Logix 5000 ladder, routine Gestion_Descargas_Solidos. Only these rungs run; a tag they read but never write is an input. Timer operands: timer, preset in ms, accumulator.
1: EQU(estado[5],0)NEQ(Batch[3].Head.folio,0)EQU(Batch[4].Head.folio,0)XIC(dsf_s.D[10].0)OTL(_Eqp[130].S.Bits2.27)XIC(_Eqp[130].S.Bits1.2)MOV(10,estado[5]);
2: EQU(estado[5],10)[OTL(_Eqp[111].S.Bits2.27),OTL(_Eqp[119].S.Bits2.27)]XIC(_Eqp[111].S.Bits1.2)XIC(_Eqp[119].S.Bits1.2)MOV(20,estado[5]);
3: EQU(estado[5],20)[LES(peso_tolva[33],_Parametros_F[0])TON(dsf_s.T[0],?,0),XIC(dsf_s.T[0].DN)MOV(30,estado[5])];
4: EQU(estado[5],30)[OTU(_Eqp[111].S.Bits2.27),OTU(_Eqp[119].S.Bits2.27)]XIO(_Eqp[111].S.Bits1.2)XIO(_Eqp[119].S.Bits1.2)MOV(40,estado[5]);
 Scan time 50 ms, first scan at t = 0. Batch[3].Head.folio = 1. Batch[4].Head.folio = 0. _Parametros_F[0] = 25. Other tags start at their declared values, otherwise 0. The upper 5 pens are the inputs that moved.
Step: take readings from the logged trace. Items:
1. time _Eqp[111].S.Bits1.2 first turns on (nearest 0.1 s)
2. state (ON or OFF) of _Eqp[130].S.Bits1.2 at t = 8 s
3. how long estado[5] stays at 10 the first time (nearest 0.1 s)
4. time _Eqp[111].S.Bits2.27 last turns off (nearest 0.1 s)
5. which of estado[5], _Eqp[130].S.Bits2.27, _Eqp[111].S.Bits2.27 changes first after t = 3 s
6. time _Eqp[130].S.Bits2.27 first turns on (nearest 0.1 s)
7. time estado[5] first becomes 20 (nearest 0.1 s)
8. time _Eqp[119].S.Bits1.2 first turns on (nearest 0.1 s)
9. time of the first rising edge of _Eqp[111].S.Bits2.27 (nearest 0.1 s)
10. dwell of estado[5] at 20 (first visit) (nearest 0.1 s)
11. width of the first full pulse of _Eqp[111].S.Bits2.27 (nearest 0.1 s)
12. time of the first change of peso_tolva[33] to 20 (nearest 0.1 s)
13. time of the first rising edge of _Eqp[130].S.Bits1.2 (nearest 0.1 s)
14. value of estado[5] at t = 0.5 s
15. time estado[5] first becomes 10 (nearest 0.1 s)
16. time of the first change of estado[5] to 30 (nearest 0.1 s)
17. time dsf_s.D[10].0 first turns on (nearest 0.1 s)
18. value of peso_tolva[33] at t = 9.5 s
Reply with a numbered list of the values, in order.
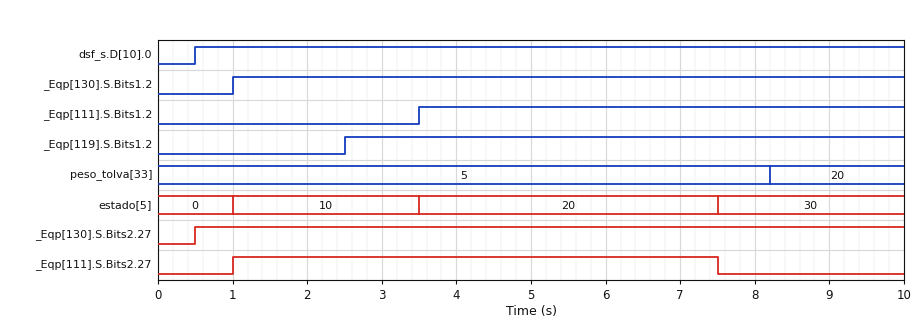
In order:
1. 3.5 s
2. ON
3. 2.5 s
4. 7.5 s
5. estado[5]
6. 0.5 s
7. 3.5 s
8. 2.5 s
9. 1.0 s
10. 4.0 s
11. 6.5 s
12. 8.2 s
13. 1.0 s
14. 0
15. 1.0 s
16. 7.5 s
17. 0.5 s
18. 20
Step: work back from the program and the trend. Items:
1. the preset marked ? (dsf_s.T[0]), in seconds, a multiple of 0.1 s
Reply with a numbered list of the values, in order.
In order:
1. 4.0 s
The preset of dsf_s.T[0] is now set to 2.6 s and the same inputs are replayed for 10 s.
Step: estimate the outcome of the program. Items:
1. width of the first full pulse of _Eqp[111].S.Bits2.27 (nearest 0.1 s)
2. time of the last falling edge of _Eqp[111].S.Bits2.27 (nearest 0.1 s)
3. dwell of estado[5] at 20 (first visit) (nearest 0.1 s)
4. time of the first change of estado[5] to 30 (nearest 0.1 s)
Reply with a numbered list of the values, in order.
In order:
1. 5.1 s
2. 6.1 s
3. 2.6 s
4. 6.1 s
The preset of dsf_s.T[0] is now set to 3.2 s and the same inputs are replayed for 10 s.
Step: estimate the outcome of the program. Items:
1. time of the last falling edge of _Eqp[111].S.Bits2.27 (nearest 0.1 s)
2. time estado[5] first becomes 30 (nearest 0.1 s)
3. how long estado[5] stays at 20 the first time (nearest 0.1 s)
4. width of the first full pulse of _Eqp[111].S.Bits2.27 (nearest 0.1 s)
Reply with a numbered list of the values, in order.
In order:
1. 6.7 s
2. 6.7 s
3. 3.2 s
4. 5.7 s
